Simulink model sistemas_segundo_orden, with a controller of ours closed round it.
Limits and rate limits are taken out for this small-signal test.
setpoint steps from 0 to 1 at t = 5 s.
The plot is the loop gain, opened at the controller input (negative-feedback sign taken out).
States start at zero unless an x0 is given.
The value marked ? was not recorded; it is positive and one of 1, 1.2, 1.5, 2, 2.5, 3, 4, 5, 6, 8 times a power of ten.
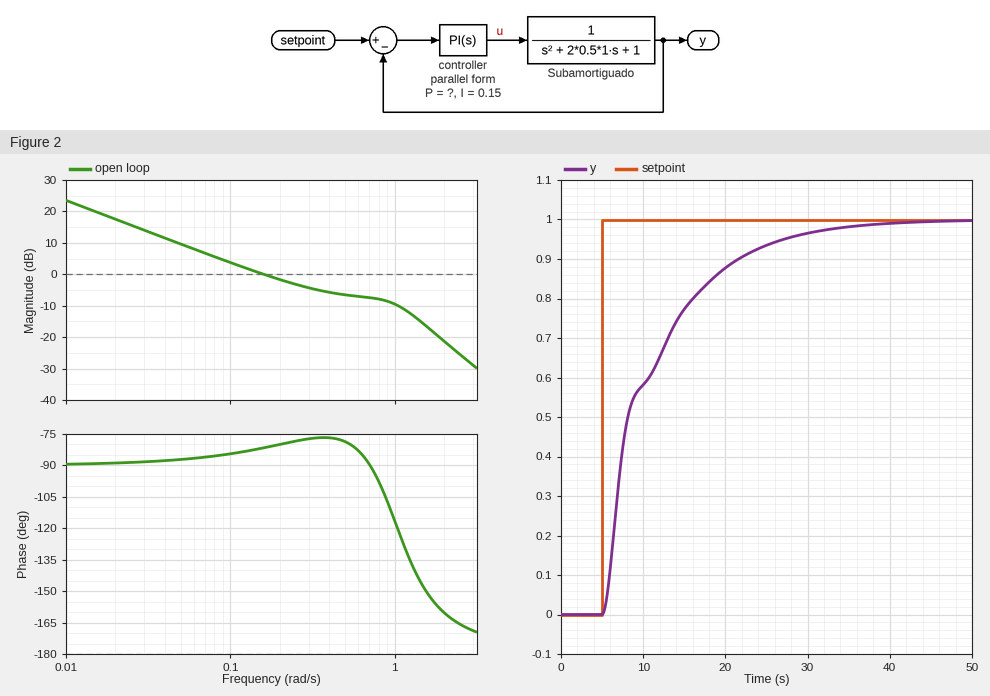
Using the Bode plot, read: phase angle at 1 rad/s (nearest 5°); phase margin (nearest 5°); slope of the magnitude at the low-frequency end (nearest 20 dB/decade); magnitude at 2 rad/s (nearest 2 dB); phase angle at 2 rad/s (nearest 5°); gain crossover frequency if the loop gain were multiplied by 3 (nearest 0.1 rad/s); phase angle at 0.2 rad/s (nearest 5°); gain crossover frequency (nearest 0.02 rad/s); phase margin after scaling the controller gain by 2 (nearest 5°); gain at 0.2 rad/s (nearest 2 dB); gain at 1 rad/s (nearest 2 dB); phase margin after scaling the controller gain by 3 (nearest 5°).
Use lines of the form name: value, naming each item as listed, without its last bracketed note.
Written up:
phase angle at 1 rad/s: -115°
phase margin: 100°
slope of the magnitude at the low-frequency end: -20 dB/decade
magnitude at 2 rad/s: -22 dB
phase angle at 2 rad/s: -160°
gain crossover frequency if the loop gain were multiplied by 3: 1.0 rad/s
phase angle at 0.2 rad/s: -80°
gain crossover frequency: 0.16 rad/s
phase margin after scaling the controller gain by 2: 105°
gain at 0.2 rad/s: -2 dB
gain at 1 rad/s: -10 dB
phase margin after scaling the controller gain by 3: 65°
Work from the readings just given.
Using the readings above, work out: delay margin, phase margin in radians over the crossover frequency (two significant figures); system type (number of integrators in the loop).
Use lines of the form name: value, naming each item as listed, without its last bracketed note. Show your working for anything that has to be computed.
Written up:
delay margin, phase margin in radians over the crossover frequency: 100 × π / 180 / 0.16 = 11 s
system type: 1
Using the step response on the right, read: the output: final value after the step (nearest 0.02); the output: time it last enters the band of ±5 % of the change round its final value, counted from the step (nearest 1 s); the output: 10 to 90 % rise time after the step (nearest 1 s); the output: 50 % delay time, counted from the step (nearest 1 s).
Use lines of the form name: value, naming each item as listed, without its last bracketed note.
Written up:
the output: final value after the step: 1.00
the output: time it last enters the band of ±5 % of the change round its final value, counted from the step: 22 s
the output: 10 to 90 % rise time after the step: 16 s
the output: 50 % delay time, counted from the step: 3 s
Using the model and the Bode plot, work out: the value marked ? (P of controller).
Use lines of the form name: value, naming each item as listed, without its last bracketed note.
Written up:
the value marked ?: 0.3
